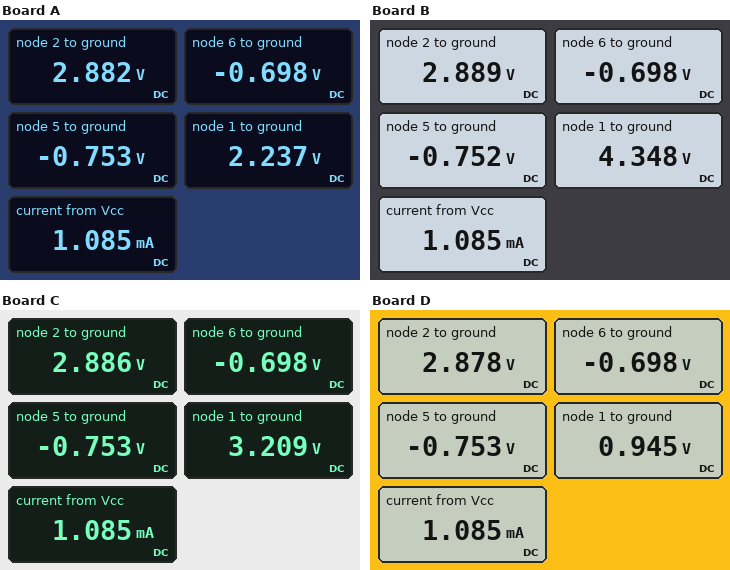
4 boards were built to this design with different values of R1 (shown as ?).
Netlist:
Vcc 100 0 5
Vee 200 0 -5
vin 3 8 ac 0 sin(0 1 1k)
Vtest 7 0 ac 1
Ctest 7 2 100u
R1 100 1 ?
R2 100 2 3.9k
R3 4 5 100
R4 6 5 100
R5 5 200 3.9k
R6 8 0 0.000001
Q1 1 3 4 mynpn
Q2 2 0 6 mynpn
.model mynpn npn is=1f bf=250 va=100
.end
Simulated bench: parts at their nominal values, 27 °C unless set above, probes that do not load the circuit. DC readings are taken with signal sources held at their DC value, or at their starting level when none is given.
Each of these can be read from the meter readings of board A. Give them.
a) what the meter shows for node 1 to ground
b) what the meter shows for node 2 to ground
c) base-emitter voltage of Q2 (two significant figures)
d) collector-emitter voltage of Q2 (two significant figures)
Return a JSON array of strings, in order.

["2.237 V", "2.882 V", "700 mV", "3.6 V"]
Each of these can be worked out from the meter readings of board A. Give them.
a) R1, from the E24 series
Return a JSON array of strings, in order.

["5.1 kΩ"]
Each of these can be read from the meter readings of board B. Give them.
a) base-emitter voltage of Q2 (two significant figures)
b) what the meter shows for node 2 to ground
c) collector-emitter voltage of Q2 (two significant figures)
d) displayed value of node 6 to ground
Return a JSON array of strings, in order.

["700 mV", "2.889 V", "3.6 V", "-0.698 V"]
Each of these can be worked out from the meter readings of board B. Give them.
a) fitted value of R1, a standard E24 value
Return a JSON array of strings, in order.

["1.2 kΩ"]
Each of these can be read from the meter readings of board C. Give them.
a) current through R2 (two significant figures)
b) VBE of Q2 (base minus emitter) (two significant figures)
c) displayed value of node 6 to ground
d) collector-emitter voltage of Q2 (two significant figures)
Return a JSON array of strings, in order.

["540 µA", "700 mV", "-0.698 V", "3.6 V"]
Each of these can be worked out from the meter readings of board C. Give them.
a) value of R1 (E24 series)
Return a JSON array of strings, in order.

["3.3 kΩ"]
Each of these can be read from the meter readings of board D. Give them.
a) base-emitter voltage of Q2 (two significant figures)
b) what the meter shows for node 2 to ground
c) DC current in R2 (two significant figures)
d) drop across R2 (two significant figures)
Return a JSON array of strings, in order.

["700 mV", "2.878 V", "540 µA", "2.1 V"]
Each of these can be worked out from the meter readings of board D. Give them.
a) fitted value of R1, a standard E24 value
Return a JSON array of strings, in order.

["7.5 kΩ"]
